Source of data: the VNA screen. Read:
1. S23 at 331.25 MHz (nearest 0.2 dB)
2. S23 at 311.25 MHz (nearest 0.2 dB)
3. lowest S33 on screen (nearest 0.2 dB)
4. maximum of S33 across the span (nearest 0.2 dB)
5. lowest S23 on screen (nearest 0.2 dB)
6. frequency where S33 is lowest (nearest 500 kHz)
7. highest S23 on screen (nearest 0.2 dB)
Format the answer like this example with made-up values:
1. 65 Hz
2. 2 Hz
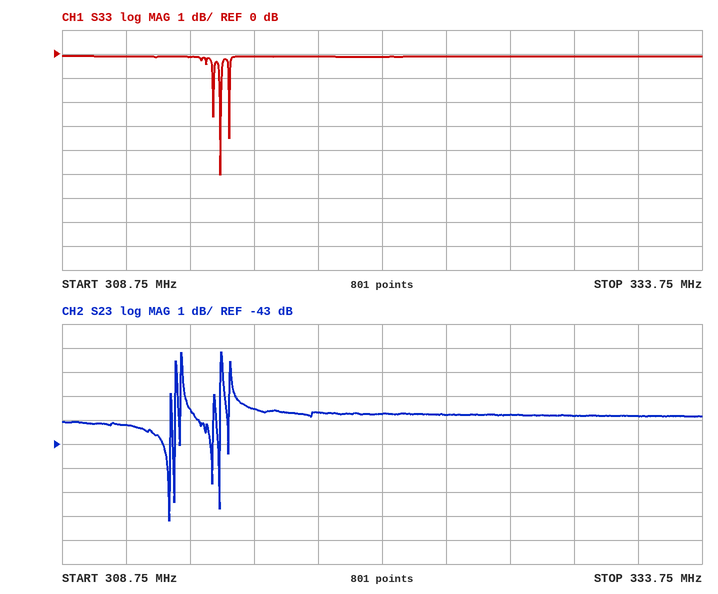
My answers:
1. -41.8 dB
2. -42.2 dB
3. -5.0 dB
4. 0.0 dB
5. -46.2 dB
6. 315.0 MHz
7. -39.2 dB
